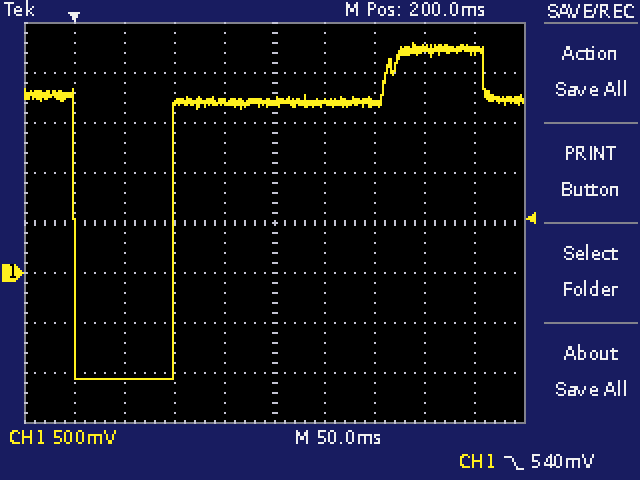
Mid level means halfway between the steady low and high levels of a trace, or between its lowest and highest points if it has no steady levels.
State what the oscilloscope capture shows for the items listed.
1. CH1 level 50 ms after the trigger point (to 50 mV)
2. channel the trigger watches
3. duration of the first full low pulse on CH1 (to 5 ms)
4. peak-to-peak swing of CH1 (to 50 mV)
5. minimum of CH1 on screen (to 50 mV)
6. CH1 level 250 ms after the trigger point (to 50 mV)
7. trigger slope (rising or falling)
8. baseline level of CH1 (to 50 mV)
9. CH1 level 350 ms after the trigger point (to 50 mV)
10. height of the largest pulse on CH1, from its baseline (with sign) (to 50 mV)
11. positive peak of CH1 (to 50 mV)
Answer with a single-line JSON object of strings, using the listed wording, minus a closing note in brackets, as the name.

{"CH1 level 50 ms after the trigger point": "-1.05 V", "channel the trigger watches": "CH1", "duration of the first full low pulse on CH1": "100 ms", "peak-to-peak swing of CH1": "3.35 V", "minimum of CH1 on screen": "-1.05 V", "CH1 level 250 ms after the trigger point": "1.70 V", "trigger slope": "falling", "baseline level of CH1": "1.70 V", "CH1 level 350 ms after the trigger point": "2.25 V", "height of the largest pulse on CH1, from its baseline (with sign)": "-2.75 V", "positive peak of CH1": "2.30 V"}
